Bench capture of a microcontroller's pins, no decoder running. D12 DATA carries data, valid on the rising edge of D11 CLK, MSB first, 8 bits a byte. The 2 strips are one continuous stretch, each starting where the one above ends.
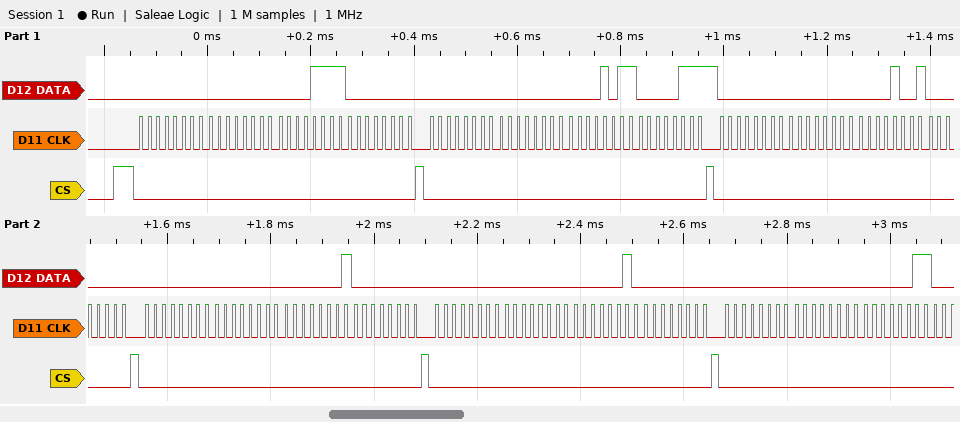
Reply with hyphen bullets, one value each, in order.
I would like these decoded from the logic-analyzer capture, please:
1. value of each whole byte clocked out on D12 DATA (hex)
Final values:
- 0x00 0x00 0x0F 0x00 0x00 0x00 0x0B 0x07 0x00 0x00 0x09 0x00 0x00 0x00 0x01 0x00 0x00 0x00 0x02 0x00 0x00 0x00 0x03
